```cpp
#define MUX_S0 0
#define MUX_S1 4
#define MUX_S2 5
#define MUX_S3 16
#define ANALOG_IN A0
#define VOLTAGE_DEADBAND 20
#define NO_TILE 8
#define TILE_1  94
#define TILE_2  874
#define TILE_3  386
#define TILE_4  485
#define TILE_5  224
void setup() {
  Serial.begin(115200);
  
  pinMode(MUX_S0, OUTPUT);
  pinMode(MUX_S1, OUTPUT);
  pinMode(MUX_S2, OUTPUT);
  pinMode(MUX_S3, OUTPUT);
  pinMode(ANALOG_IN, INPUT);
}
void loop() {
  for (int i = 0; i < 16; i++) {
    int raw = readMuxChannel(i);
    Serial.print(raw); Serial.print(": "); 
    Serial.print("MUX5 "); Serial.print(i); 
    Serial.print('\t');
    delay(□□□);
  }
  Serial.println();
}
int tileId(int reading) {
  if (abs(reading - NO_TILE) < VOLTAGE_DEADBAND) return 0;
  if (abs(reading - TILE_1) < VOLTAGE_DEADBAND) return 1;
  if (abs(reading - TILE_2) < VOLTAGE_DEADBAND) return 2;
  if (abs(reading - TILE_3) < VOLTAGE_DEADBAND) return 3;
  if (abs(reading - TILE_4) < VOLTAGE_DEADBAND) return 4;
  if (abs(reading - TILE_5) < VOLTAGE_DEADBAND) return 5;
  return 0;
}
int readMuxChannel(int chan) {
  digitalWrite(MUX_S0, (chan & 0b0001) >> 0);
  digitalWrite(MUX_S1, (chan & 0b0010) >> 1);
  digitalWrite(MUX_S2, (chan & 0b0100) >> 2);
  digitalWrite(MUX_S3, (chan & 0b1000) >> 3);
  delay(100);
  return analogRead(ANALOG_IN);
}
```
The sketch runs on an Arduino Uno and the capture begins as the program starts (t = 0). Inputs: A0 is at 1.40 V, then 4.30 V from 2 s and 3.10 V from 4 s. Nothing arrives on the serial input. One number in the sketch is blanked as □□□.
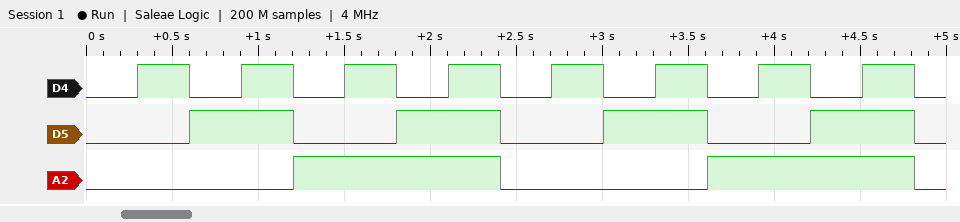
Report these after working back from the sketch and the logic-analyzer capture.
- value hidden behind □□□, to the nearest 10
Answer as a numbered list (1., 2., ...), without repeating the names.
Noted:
1. 50
